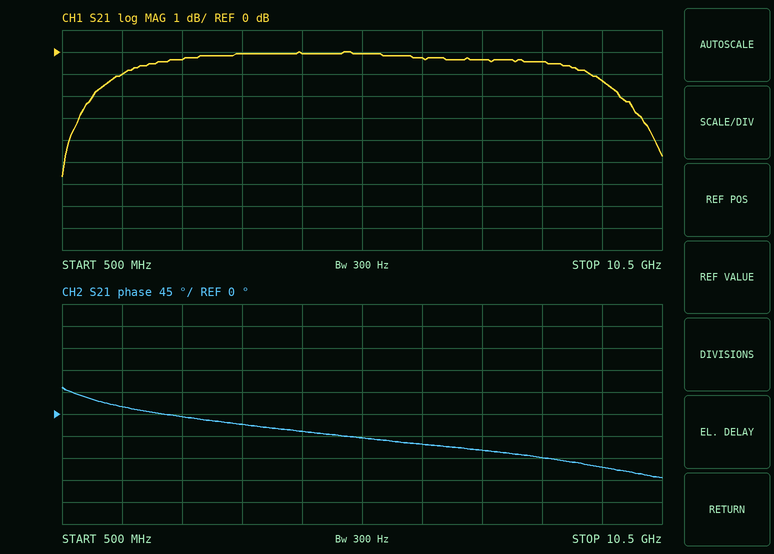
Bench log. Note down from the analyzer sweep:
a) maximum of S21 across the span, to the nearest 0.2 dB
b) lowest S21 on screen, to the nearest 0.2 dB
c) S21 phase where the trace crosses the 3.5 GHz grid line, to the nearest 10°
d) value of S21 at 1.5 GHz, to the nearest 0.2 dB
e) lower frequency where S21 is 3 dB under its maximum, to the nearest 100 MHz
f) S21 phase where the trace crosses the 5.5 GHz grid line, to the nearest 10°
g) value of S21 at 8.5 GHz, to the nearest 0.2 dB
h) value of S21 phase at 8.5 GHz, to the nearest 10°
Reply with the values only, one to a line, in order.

0.0 dB
-5.6 dB
-20°
-1.0 dB
800 MHz
-50°
-0.4 dB
-90°
